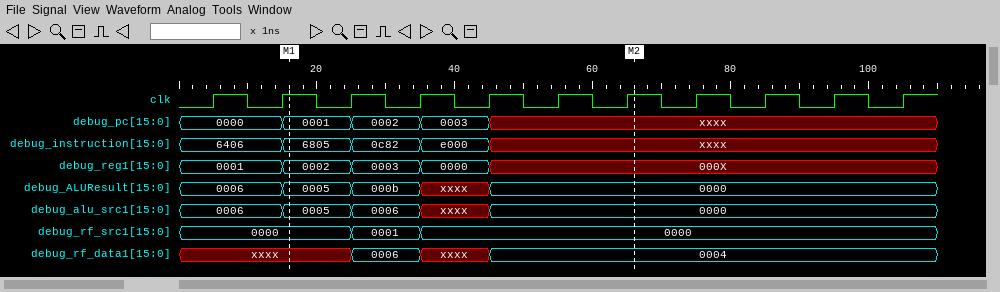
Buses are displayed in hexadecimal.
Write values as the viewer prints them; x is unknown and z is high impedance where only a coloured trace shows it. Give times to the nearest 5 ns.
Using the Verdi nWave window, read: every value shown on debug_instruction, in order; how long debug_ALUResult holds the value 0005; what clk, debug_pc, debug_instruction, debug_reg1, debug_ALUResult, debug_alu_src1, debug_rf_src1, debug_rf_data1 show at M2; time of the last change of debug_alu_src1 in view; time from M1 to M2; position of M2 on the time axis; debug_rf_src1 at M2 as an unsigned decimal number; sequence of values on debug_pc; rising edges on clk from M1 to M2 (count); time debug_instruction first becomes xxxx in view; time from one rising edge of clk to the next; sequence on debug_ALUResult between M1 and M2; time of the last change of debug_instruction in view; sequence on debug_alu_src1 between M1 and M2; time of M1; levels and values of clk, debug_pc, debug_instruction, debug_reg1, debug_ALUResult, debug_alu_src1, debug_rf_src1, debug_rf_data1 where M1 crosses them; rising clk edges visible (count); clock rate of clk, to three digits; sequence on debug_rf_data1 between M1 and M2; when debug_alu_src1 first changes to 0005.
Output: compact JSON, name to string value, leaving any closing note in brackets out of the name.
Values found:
{"every value shown on debug_instruction, in order": "6406, 6805, 0c82, e000, xxxx", "how long debug_ALUResult holds the value 0005": "10 ns", "what clk, debug_pc, debug_instruction, debug_reg1, debug_ALUResult, debug_alu_src1, debug_rf_src1, debug_rf_data1 show at M2": "clk=1, debug_pc=xxxx, debug_instruction=xxxx, debug_reg1=000X, debug_ALUResult=0000, debug_alu_src1=0000, debug_rf_src1=0000, debug_rf_data1=0004", "time of the last change of debug_alu_src1 in view": "45 ns", "time from M1 to M2": "50 ns", "position of M2 on the time axis": "65 ns", "debug_rf_src1 at M2 as an unsigned decimal number": "0", "sequence of values on debug_pc": "0000, 0001, 0002, 0003, xxxx", "rising edges on clk from M1 to M2": "5", "time debug_instruction first becomes xxxx in view": "45 ns", "time from one rising edge of clk to the next": "10 ns", "sequence on debug_ALUResult between M1 and M2": "0005, 000b, xxxx, 0000", "time of the last change of debug_instruction in view": "45 ns", "sequence on debug_alu_src1 between M1 and M2": "0005, 0006, xxxx, 0000", "time of M1": "15 ns", "levels and values of clk, debug_pc, debug_instruction, debug_reg1, debug_ALUResult, debug_alu_src1, debug_rf_src1, debug_rf_data1 where M1 crosses them": "clk=1, debug_pc=0001, debug_instruction=6805, debug_reg1=0002, debug_ALUResult=0005, debug_alu_src1=0005, debug_rf_src1=0000, debug_rf_data1=xxxx", "rising clk edges visible": "11", "clock rate of clk, to three digits": "100 MHz", "sequence on debug_rf_data1 between M1 and M2": "xxxx, 0006, xxxx, 0004", "when debug_alu_src1 first changes to 0005": "15 ns"}
